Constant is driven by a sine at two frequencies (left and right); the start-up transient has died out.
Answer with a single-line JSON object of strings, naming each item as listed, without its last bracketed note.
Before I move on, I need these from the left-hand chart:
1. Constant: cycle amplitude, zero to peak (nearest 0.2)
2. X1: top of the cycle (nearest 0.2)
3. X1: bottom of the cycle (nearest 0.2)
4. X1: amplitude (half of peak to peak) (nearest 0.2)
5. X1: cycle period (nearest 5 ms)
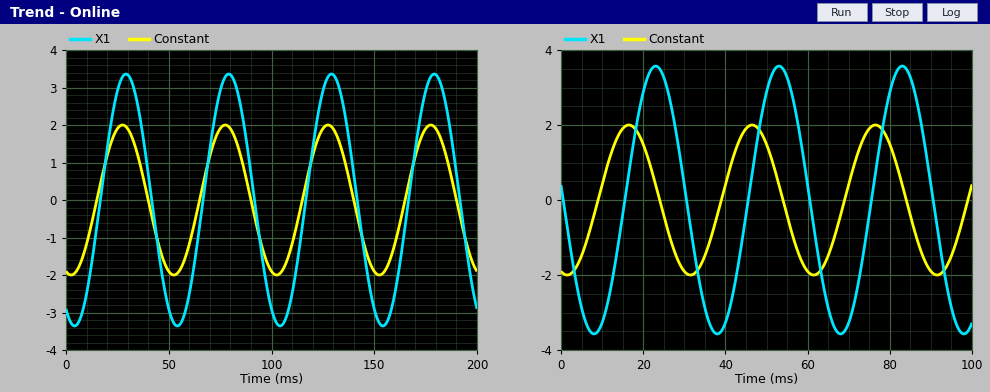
{"Constant: cycle amplitude, zero to peak": "2.0", "X1: top of the cycle": "3.4", "X1: bottom of the cycle": "-3.4", "X1: amplitude (half of peak to peak)": "3.4", "X1: cycle period": "50 ms"}
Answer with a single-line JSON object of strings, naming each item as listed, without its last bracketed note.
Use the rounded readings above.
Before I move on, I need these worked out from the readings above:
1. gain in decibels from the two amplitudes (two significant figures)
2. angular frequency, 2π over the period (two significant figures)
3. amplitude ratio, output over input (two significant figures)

{"gain in decibels from the two amplitudes": "4.6 dB", "angular frequency, 2π over the period": "0.13 rad/ms", "amplitude ratio, output over input": "1.7"}
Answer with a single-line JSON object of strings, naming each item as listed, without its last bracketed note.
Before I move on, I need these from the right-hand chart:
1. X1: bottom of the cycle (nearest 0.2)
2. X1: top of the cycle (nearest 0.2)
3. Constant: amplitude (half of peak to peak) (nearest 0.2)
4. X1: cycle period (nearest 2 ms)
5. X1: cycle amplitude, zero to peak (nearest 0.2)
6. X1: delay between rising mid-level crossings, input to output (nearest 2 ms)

{"X1: bottom of the cycle": "-3.6", "X1: top of the cycle": "3.6", "Constant: amplitude (half of peak to peak)": "2.0", "X1: cycle period": "30 ms", "X1: cycle amplitude, zero to peak": "3.6", "X1: delay between rising mid-level crossings, input to output": "6 ms"}
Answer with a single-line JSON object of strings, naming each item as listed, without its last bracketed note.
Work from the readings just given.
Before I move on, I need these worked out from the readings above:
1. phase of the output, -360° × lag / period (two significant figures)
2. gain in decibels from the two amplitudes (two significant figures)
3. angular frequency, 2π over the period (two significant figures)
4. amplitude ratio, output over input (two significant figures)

{"phase of the output, -360° × lag / period": "-72°", "gain in decibels from the two amplitudes": "5.1 dB", "angular frequency, 2π over the period": "0.21 rad/ms", "amplitude ratio, output over input": "1.8"}
